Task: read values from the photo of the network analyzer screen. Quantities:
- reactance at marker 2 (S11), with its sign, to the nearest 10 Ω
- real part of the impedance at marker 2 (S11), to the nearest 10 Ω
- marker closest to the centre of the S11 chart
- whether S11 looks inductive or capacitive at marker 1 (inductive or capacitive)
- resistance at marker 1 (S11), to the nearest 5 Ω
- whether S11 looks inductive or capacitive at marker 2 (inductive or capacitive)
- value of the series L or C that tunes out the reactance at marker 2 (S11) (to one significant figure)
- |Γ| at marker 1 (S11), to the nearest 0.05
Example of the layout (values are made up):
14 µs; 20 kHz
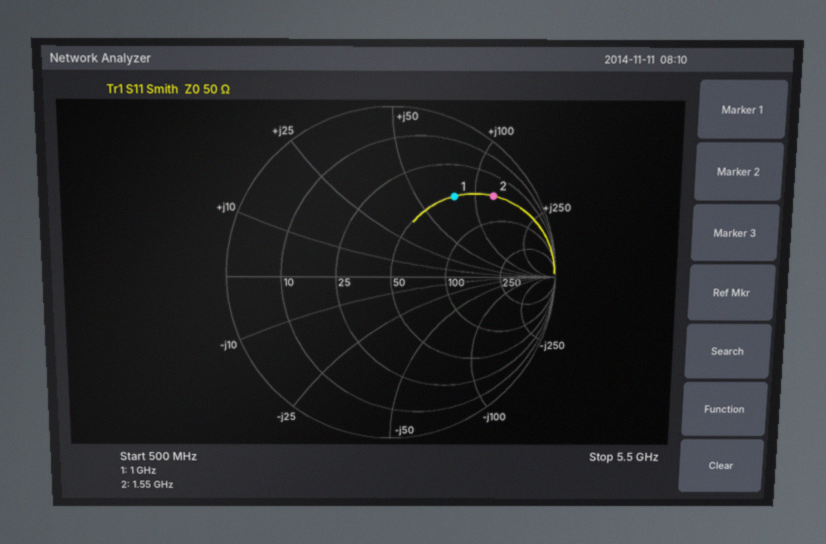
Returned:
+130 Ω; 50 Ω; marker 1; inductive; 50 Ω; inductive; 800 fF; 0.60
